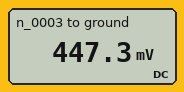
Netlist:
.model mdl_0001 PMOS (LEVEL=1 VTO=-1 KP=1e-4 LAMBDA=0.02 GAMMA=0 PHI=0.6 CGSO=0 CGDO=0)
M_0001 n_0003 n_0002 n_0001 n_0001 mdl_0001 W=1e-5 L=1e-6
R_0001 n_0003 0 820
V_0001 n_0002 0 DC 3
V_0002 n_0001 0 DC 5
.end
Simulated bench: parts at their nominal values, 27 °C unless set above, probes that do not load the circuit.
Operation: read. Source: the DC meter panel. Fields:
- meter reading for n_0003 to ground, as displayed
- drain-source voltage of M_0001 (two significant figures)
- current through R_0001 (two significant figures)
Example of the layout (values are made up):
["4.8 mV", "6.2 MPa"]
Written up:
["447.3 mV", "-4.6 V", "550 µA"]
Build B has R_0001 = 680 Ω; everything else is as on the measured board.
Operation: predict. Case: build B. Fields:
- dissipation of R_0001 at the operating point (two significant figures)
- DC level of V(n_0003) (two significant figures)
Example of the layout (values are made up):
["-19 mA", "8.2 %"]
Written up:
["200 µW", "370 mV"]
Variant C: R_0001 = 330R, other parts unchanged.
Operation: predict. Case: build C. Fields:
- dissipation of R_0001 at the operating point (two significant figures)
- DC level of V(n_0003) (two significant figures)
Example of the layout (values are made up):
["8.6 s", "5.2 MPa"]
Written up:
["99 µW", "180 mV"]
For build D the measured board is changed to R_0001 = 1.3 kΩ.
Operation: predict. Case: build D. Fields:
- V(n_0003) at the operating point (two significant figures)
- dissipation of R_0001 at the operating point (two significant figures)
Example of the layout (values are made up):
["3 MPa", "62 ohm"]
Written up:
["710 mV", "380 µW"]
